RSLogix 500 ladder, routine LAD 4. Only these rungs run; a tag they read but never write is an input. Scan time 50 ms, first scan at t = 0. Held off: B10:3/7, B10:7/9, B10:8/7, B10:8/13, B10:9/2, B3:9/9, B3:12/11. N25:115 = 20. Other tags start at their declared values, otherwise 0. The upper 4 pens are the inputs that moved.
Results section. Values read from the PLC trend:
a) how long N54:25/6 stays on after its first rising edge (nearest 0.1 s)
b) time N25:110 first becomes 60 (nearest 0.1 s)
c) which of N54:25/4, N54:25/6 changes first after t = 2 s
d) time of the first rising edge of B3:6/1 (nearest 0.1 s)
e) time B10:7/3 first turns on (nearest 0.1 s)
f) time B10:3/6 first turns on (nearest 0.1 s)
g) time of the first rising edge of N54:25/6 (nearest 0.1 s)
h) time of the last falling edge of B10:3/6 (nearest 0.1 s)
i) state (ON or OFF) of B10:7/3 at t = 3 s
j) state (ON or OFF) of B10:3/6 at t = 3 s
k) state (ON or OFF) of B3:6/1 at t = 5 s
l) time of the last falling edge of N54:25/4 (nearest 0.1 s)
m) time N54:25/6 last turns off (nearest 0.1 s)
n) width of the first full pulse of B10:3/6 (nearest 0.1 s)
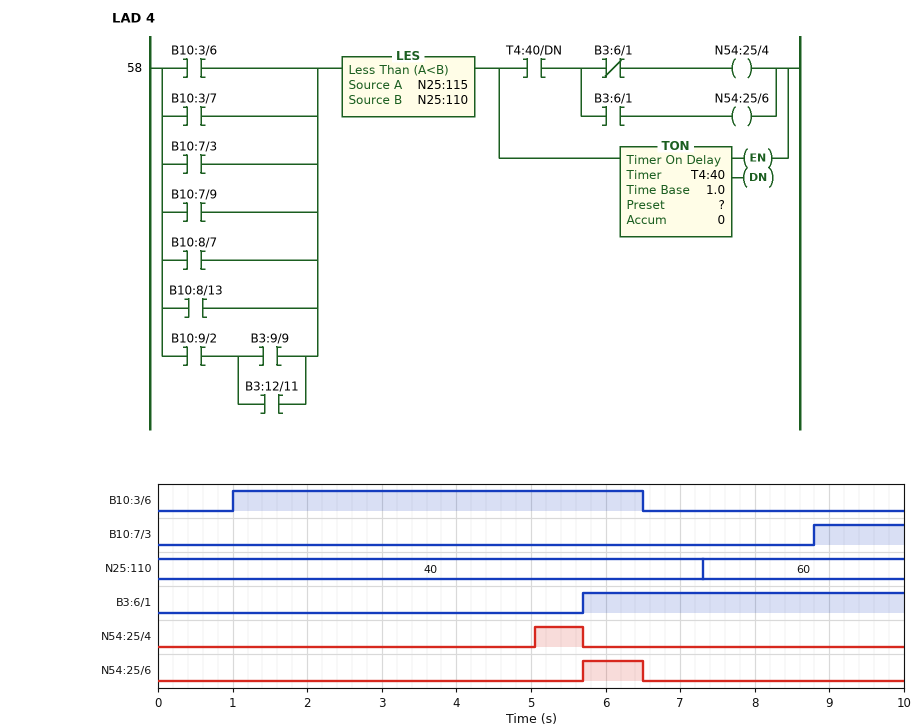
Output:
0.8 s
7.3 s
N54:25/4
5.7 s
8.8 s
1.0 s
5.7 s
6.5 s
OFF
ON
OFF
5.7 s
6.5 s
5.5 s
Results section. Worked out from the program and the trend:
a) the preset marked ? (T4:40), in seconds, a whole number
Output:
4 s
